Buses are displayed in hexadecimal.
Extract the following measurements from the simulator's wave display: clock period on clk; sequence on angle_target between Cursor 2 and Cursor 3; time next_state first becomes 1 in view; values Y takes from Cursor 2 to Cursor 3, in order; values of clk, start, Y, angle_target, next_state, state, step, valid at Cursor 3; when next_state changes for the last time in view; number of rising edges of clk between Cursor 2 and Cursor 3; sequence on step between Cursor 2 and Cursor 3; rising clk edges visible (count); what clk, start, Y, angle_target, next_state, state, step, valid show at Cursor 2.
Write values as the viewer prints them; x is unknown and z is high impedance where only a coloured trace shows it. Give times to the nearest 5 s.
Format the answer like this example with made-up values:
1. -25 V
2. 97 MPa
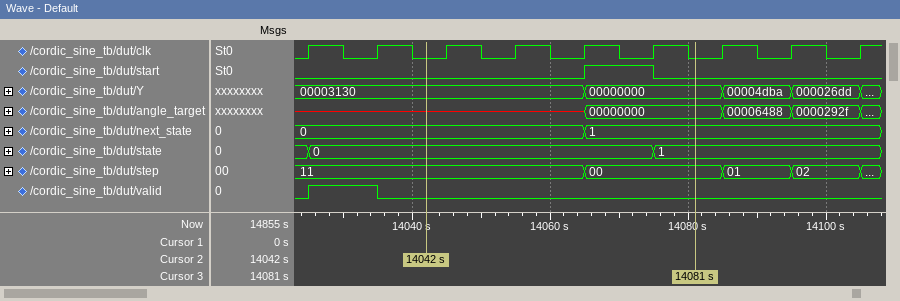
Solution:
1. 10 s
2. x, 00000000
3. 14065 s
4. 00003130, 00000000
5. clk=0, start=0, Y=00000000, angle_target=00000000, next_state=1, state=1, step=00, valid=0
6. 14065 s
7. 4
8. 11, 00
9. 9
10. clk=0, start=0, Y=00003130, angle_target=x, next_state=0, state=0, step=11, valid=0
